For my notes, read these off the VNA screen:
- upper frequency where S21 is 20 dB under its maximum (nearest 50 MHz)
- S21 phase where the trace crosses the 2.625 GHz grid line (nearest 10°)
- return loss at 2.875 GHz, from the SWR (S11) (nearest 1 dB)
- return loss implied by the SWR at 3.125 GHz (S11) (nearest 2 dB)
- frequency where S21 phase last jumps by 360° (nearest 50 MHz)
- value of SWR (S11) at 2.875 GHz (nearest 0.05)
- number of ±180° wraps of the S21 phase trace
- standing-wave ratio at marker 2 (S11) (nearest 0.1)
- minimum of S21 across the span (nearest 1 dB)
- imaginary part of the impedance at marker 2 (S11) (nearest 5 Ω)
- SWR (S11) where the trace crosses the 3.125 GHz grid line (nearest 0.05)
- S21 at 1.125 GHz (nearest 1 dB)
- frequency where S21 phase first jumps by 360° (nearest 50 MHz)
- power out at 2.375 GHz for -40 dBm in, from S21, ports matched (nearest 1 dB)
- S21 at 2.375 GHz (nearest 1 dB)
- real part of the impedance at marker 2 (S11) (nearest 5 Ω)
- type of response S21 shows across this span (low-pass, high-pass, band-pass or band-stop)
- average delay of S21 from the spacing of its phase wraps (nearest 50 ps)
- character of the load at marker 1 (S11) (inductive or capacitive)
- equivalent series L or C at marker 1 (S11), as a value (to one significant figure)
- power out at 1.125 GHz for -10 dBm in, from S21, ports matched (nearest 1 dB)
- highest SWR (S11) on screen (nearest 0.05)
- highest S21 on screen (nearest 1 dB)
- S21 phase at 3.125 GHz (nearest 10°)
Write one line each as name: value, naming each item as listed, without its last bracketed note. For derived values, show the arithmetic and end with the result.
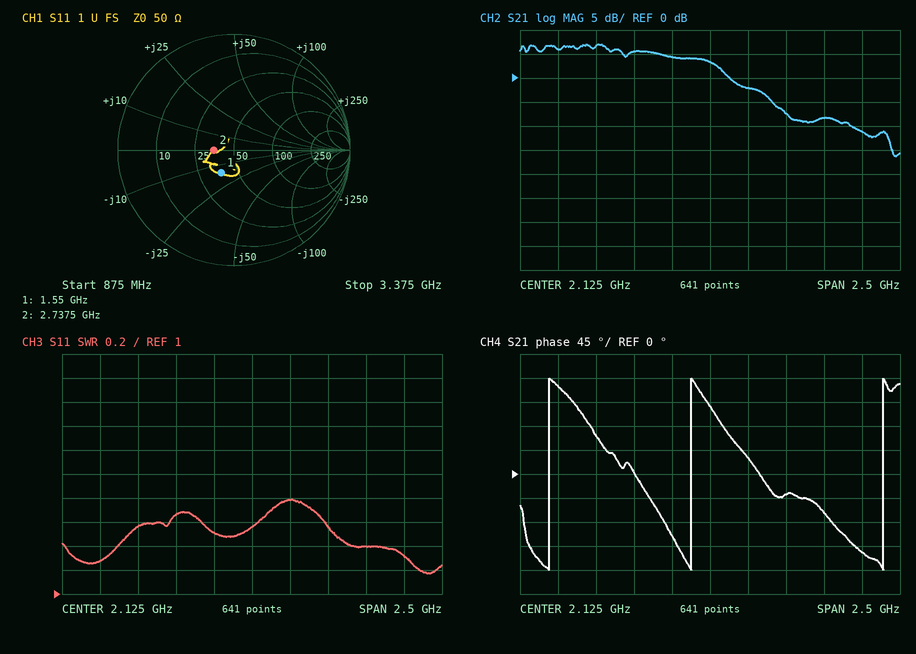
upper frequency where S21 is 20 dB under its maximum: 3.30 GHz
S21 phase where the trace crosses the 2.625 GHz grid line: -40°
return loss at 2.875 GHz, from the SWR (S11): −20 log10((1.4 − 1)/(1.4 + 1)) ≈ 16 dB
return loss implied by the SWR at 3.125 GHz (S11): −20 log10((1.3 − 1)/(1.3 + 1)) ≈ 18 dB
frequency where S21 phase last jumps by 360°: 3.25 GHz
value of SWR (S11) at 2.875 GHz: 1.40
number of ±180° wraps of the S21 phase trace: 3
standing-wave ratio at marker 2 (S11): 1.4
minimum of S21 across the span: -16 dB
imaginary part of the impedance at marker 2 (S11): 0 Ω
SWR (S11) where the trace crosses the 3.125 GHz grid line: 1.30
S21 at 1.125 GHz: 6 dB
frequency where S21 phase first jumps by 360°: 1.05 GHz
power out at 2.375 GHz for -40 dBm in, from S21, ports matched: -40 dBm + (-2 dB) = -42 dBm
S21 at 2.375 GHz: -2 dB
real part of the impedance at marker 2 (S11): 35 Ω
type of response S21 shows across this span: low-pass
average delay of S21 from the spacing of its phase wraps: 2 cycles / (3.25 GHz − 1.05 GHz) ≈ 909 ps, so 900 ps to the nearest 50 ps
character of the load at marker 1 (S11): capacitive
equivalent series L or C at marker 1 (S11), as a value: C = 1/(2π × 1.55 GHz × 15 Ω) ≈ 7 pF
power out at 1.125 GHz for -10 dBm in, from S21, ports matched: -10 dBm + (6 dB) = -4 dBm
highest SWR (S11) on screen: 1.80
highest S21 on screen: 7 dB
S21 phase at 3.125 GHz: -150°
